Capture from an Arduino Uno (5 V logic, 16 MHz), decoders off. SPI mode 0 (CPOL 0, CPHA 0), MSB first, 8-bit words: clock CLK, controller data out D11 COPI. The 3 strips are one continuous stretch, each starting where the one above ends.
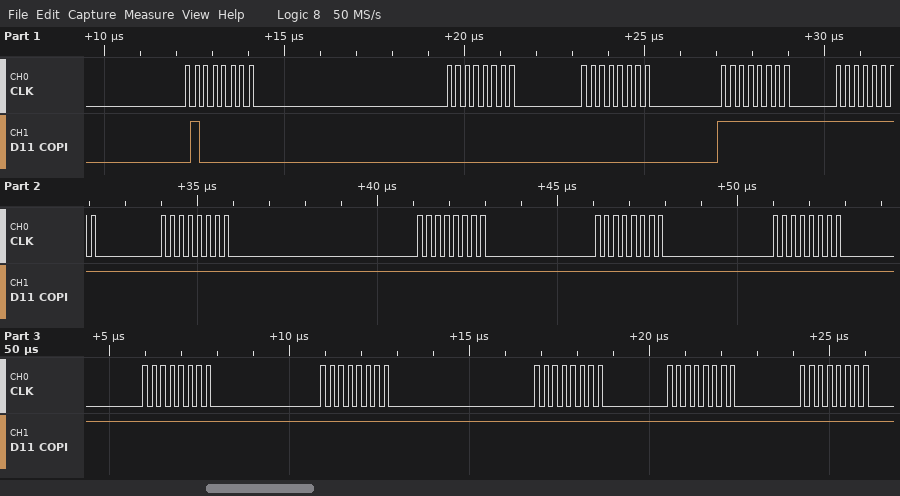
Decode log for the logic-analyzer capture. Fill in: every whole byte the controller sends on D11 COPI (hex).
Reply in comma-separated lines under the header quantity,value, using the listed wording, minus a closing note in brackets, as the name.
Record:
quantity,value
every whole byte the controller sends on D11 COPI,40 00 00 FF FF FF FF FF FF FF FF FF FF FF
